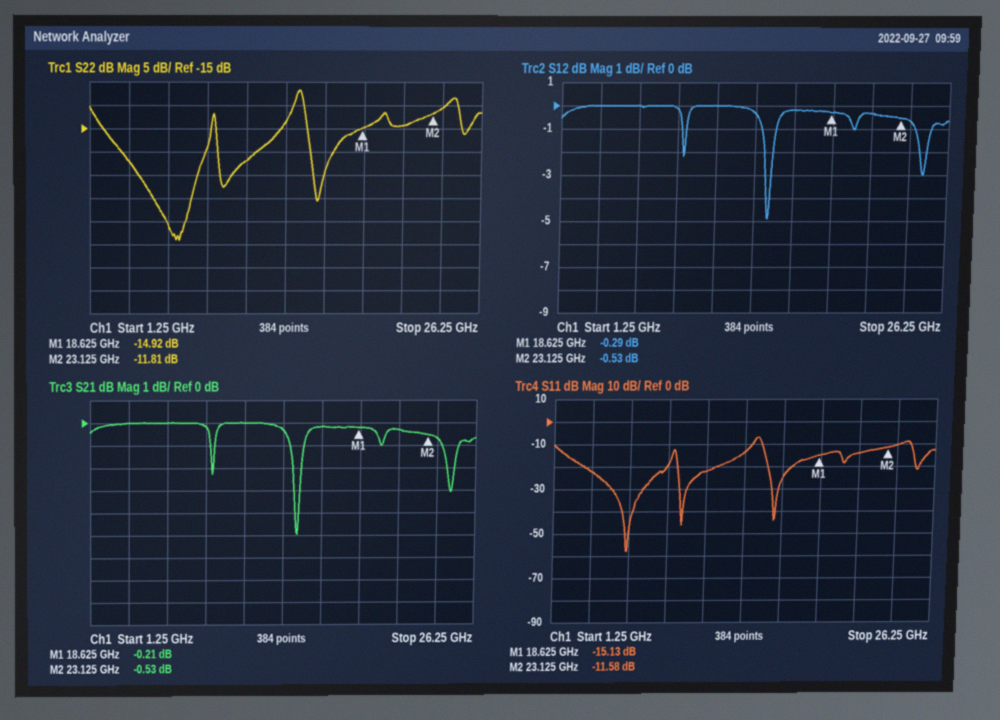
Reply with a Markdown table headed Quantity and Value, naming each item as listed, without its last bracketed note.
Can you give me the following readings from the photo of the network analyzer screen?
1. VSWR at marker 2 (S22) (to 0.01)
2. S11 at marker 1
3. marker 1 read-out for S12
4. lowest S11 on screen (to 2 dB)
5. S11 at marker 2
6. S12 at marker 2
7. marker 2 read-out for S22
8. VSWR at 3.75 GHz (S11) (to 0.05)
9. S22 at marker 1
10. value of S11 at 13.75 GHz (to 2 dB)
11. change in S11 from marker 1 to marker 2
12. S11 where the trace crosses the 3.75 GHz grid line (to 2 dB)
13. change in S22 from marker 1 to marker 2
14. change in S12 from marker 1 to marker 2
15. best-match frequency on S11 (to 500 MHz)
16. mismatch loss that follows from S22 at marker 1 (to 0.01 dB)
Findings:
| Quantity | Value |
|---|---|
| VSWR at marker 2 (S22) | 1.69 |
| S11 at marker 1 | -15.13 dB |
| marker 1 read-out for S12 | -0.29 dB |
| lowest S11 on screen | -58 dB |
| S11 at marker 2 | -11.58 dB |
| S12 at marker 2 | -0.53 dB |
| marker 2 read-out for S22 | -11.81 dB |
| VSWR at 3.75 GHz (S11) | 1.15 |
| S22 at marker 1 | -14.92 dB |
| value of S11 at 13.75 GHz | -14 dB |
| change in S11 from marker 1 to marker 2 | 3.55 dB |
| S11 where the trace crosses the 3.75 GHz grid line | -22 dB |
| change in S22 from marker 1 to marker 2 | 3.11 dB |
| change in S12 from marker 1 to marker 2 | -0.24 dB |
| best-match frequency on S11 | 6.0 GHz |
| mismatch loss that follows from S22 at marker 1 | 0.14 dB |
